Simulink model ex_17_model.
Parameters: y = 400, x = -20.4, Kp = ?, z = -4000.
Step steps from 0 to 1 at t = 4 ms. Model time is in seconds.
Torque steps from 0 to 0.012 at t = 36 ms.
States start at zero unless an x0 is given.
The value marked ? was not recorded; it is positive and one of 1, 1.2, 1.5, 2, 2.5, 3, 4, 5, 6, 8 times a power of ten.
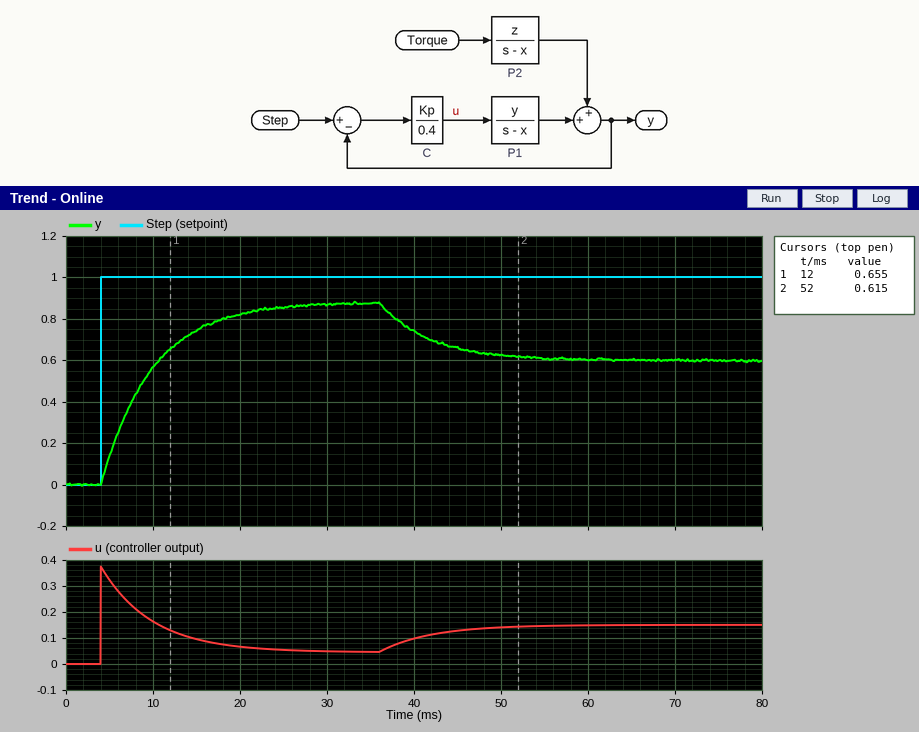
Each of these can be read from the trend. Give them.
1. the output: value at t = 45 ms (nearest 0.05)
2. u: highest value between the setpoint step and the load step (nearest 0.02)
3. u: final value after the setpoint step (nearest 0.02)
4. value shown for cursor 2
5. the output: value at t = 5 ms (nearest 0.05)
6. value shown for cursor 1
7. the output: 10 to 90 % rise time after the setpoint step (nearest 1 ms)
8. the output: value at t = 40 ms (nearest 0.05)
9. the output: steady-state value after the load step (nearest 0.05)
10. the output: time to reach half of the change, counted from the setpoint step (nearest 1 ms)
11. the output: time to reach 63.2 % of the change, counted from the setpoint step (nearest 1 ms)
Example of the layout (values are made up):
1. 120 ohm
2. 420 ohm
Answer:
1. 0.65
2. 0.38
3. 0.04
4. 0.615
5. 0.15
6. 0.655
7. 13 ms
8. 0.75
9. 0.60
10. 4 ms
11. 6 ms
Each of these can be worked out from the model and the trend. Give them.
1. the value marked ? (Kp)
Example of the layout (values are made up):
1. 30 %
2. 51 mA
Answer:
1. 0.15
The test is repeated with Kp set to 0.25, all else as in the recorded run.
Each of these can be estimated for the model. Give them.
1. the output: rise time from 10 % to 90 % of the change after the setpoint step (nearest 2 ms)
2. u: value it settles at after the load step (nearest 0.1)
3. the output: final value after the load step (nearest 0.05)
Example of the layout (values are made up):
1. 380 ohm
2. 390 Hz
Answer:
1. 8 ms
2. 0.2
3. 0.75
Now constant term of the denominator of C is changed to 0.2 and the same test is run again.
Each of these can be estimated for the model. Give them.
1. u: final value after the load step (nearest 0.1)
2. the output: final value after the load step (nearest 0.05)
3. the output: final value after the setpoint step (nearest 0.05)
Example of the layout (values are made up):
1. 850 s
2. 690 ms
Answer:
1. 0.2
2. 0.80
3. 0.95
